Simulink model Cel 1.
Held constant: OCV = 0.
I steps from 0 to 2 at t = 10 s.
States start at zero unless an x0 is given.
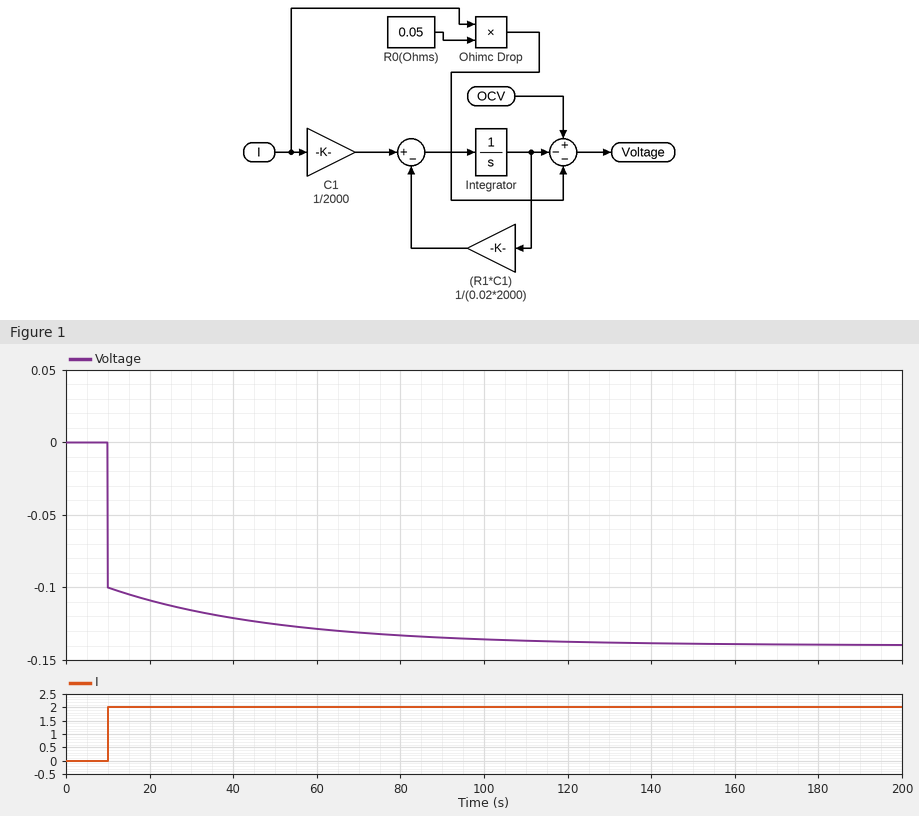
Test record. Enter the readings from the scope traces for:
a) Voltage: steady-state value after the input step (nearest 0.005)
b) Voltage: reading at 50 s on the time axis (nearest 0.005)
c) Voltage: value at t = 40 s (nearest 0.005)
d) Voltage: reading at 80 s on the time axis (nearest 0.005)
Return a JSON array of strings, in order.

["-0.140", "-0.125", "-0.120", "-0.135"]
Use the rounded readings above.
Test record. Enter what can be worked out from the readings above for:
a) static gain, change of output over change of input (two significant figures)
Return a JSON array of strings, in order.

["-0.070"]
